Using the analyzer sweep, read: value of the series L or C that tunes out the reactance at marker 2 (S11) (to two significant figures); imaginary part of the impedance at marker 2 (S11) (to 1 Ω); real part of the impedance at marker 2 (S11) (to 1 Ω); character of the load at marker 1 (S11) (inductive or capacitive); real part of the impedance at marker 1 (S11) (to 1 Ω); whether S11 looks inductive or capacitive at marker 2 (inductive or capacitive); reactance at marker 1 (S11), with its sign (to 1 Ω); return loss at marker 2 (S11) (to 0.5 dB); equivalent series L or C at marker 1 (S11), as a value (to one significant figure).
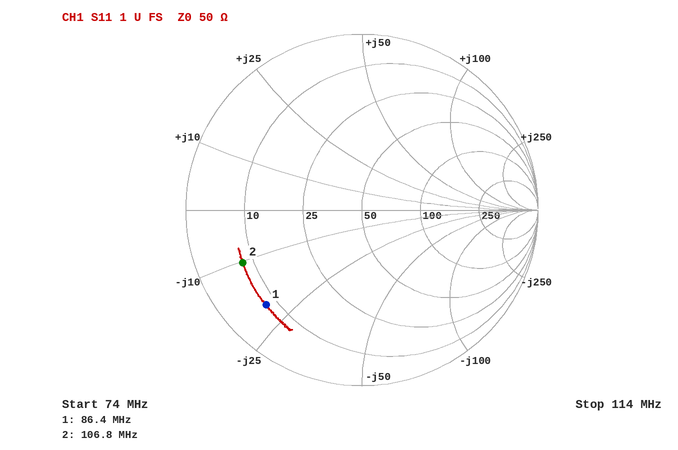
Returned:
15 nH
-10 Ω
8 Ω
capacitive
8 Ω
capacitive
-20 Ω
2.5 dB
90 pF
